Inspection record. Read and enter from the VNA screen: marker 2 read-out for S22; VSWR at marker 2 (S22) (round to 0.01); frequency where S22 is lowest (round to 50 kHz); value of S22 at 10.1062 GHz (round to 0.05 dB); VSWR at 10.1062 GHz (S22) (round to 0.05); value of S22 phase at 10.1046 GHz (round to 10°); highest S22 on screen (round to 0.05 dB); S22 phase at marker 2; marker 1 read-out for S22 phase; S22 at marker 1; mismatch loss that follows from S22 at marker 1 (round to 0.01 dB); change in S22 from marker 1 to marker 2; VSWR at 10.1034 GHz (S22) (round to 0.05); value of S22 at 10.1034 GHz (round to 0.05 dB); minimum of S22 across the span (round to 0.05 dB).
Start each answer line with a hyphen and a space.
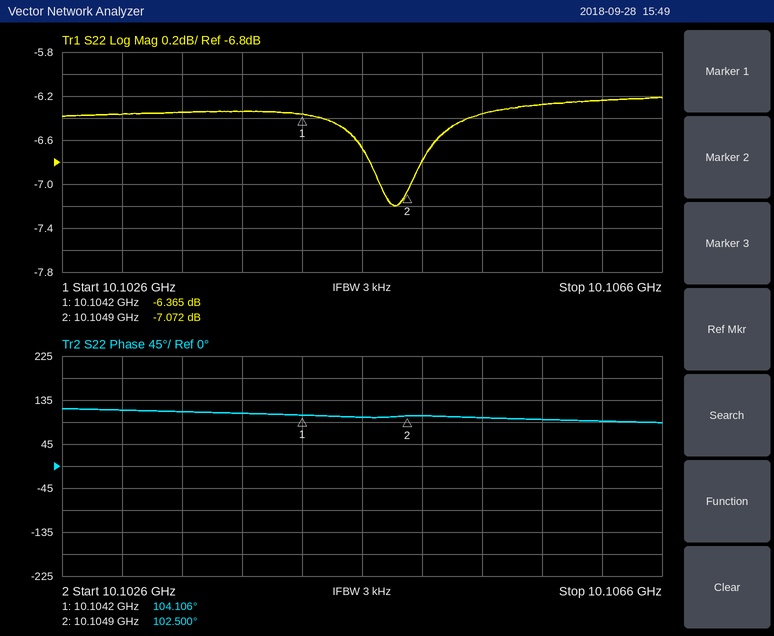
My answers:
- -7.072 dB
- 2.59
- 10.10480 GHz
- -6.25 dB
- 2.90
- 100°
- -6.20 dB
- 102.500°
- 104.106°
- -6.365 dB
- 1.14 dB
- -0.707 dB
- 2.85
- -6.35 dB
- -7.20 dB
